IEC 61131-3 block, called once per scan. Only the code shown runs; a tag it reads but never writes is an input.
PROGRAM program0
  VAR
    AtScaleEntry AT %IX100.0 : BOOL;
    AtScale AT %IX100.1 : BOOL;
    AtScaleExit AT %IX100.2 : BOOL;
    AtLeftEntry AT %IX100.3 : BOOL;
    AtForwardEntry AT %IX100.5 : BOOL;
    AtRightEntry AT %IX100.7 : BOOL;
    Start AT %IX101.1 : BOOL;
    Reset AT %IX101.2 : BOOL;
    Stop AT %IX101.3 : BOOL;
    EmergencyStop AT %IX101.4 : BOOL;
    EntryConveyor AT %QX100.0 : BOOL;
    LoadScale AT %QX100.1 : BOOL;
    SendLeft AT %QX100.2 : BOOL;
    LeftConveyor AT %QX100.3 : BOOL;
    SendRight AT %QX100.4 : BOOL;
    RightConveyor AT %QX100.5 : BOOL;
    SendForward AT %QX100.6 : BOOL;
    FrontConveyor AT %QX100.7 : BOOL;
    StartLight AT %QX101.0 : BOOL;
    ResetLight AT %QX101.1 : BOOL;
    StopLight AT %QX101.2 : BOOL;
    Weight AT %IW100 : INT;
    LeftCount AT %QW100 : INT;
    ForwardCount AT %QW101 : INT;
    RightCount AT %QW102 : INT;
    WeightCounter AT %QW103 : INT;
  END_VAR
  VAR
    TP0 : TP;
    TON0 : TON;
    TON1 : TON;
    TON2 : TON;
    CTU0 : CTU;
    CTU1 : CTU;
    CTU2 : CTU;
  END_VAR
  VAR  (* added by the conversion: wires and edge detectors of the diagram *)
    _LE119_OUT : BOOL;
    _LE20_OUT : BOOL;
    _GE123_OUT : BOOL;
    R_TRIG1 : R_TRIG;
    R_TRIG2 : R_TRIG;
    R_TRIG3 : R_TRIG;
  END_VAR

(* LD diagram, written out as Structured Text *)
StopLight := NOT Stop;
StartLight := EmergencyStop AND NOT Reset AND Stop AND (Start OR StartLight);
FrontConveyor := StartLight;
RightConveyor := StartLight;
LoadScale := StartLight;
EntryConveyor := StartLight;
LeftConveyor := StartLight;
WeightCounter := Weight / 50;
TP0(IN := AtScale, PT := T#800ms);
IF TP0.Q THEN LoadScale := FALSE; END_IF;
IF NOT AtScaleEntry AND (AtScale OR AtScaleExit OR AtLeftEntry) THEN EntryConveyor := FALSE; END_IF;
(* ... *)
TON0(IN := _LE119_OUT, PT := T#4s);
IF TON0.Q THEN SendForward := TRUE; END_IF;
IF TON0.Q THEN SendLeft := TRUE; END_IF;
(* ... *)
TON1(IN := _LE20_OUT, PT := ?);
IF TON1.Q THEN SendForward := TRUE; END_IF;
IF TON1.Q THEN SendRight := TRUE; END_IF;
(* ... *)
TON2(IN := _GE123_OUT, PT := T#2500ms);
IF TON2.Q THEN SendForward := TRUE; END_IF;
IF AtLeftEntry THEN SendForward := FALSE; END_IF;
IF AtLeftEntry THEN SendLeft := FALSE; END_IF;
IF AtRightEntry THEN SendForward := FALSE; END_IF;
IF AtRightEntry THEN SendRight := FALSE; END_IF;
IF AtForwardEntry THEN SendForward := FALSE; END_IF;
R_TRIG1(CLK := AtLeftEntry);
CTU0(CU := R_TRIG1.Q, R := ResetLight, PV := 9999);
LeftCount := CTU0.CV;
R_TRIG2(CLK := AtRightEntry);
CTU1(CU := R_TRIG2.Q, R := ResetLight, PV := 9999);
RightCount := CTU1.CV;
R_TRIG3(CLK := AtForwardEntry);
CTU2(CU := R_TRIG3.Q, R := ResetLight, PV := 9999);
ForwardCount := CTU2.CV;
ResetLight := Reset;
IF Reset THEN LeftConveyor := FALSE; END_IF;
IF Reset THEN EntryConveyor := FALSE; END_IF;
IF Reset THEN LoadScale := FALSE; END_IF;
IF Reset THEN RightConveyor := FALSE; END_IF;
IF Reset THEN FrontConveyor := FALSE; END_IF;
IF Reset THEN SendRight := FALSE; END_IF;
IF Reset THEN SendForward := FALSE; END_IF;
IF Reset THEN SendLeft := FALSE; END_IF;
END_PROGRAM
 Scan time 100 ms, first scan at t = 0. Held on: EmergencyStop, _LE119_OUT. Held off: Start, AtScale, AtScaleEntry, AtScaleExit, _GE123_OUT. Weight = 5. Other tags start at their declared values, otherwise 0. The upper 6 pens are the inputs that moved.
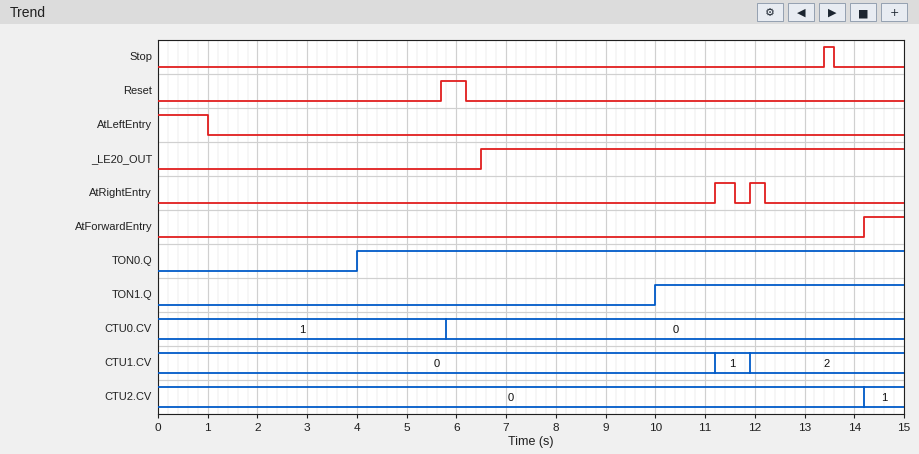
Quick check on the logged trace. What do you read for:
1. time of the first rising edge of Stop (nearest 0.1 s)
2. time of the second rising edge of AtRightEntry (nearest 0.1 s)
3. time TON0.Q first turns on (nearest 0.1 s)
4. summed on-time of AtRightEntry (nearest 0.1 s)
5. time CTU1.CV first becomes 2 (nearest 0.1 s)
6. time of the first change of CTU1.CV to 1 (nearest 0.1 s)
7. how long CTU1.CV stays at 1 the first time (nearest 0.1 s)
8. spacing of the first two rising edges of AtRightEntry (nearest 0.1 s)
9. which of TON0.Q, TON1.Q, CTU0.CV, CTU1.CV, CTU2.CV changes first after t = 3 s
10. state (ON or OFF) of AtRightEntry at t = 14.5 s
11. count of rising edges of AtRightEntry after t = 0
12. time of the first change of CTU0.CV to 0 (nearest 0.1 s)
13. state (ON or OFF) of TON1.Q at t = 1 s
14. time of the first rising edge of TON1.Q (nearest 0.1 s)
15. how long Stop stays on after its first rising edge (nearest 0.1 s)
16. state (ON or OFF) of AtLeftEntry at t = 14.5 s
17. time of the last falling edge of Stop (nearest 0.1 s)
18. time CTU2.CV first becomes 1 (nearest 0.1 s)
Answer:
13.4 s
11.9 s
4.0 s
0.7 s
11.9 s
11.2 s
0.7 s
0.7 s
TON0.Q
OFF
2
5.8 s
OFF
10.0 s
0.2 s
OFF
13.6 s
14.2 s
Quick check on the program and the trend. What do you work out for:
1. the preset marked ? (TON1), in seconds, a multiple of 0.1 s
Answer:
3.5 s
